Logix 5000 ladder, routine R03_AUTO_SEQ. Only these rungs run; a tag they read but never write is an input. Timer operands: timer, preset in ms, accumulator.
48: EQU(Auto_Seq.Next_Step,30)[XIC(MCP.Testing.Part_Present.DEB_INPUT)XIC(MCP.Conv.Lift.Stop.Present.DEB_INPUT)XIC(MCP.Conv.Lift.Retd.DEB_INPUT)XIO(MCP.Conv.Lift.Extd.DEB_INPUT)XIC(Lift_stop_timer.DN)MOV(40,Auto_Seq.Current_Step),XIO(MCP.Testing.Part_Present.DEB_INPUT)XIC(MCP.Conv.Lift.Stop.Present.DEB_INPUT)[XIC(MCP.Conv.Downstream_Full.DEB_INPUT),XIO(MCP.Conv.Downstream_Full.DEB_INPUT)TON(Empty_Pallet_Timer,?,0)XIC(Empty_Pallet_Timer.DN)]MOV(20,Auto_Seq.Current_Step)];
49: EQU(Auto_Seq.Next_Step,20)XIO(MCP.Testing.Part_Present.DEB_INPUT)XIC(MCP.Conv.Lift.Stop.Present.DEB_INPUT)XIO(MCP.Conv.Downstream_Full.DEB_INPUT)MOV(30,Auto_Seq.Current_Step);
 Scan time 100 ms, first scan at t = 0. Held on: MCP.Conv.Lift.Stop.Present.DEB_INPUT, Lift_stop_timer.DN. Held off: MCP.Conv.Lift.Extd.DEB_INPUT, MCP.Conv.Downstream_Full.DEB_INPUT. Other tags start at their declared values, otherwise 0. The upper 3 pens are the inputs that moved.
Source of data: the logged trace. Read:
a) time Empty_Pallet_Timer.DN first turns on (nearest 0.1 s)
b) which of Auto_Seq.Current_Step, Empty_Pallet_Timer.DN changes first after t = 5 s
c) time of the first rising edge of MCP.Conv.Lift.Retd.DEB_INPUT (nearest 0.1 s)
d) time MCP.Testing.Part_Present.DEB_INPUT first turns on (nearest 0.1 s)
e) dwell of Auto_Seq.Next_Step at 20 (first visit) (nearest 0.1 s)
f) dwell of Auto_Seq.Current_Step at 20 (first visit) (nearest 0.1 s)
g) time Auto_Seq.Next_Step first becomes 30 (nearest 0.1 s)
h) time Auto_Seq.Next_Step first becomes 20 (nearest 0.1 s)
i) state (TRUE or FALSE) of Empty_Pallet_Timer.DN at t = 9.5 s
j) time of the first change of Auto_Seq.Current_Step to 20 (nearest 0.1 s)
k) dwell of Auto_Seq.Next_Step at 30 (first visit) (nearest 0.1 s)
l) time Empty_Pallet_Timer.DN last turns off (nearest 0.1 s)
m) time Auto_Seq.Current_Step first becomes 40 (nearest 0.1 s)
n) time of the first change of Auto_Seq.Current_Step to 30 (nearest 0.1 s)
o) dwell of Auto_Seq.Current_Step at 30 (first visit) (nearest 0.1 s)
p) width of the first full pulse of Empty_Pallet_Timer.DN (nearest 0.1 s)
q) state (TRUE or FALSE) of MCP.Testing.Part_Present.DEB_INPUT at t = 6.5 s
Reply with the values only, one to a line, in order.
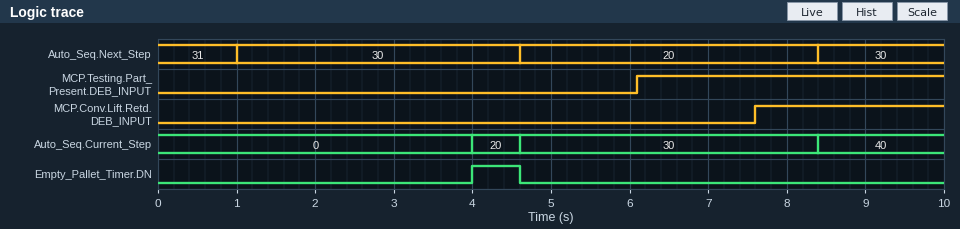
4.0 s
Auto_Seq.Current_Step
7.6 s
6.1 s
3.8 s
0.6 s
1.0 s
4.6 s
FALSE
4.0 s
3.6 s
4.6 s
8.4 s
4.6 s
3.8 s
0.6 s
TRUE
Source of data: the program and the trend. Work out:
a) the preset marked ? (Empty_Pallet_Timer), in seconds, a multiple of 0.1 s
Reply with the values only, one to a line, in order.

3.0 s
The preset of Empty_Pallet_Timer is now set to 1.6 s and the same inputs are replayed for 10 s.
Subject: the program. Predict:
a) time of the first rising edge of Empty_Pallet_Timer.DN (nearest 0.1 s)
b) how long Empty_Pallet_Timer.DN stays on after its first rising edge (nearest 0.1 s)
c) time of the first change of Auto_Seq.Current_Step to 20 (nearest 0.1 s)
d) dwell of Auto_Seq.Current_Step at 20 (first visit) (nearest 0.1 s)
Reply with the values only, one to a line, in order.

2.6 s
2.0 s
2.6 s
2.0 s
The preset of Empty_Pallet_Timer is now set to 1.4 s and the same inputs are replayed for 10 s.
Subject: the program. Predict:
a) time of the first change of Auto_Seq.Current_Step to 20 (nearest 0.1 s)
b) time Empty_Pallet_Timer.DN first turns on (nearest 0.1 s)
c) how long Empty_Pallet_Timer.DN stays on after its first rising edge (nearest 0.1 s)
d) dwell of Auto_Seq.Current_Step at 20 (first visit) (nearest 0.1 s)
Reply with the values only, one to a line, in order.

2.4 s
2.4 s
2.2 s
2.2 s
